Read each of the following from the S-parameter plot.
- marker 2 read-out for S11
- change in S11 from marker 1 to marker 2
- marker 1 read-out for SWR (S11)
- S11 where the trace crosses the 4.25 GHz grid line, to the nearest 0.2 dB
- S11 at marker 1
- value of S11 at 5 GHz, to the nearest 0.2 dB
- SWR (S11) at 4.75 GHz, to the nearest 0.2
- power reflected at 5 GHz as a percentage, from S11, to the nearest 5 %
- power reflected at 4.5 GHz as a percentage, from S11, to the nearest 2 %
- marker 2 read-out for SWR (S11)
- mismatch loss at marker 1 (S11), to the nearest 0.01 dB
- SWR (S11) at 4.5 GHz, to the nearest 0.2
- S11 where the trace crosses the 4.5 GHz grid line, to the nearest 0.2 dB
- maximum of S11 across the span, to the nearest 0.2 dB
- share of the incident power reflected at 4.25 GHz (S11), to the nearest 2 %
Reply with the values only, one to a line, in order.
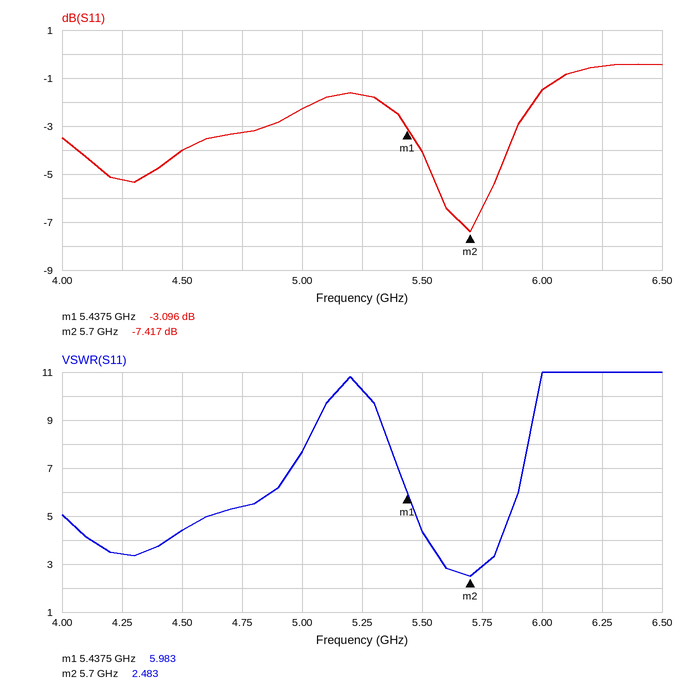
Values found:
-7.417 dB
-4.321 dB
5.983
-5.2 dB
-3.096 dB
-2.2 dB
5.4
60 %
40 %
2.483
2.93 dB
4.4
-4.0 dB
-0.4 dB
30 %
